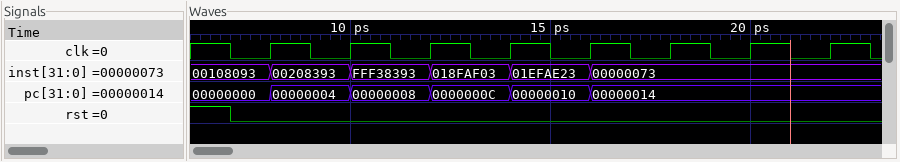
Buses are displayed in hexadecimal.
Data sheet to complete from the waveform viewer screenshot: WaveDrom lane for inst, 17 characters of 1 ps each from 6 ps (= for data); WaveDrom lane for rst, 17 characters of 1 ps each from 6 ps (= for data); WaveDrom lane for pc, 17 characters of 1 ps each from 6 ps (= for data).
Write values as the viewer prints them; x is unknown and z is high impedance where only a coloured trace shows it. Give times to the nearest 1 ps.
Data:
{name: 'inst', wave: '=.=.=.=.=.=......', data: '00108093 00208393 FFF38393 018FAF03 01EFAE23 00000073'}
{name: 'rst', wave: '10...............'}
{name: 'pc', wave: '=.=.=.=.=.=......', data: '00000000 00000004 00000008 0000000C 00000010 00000014'}
